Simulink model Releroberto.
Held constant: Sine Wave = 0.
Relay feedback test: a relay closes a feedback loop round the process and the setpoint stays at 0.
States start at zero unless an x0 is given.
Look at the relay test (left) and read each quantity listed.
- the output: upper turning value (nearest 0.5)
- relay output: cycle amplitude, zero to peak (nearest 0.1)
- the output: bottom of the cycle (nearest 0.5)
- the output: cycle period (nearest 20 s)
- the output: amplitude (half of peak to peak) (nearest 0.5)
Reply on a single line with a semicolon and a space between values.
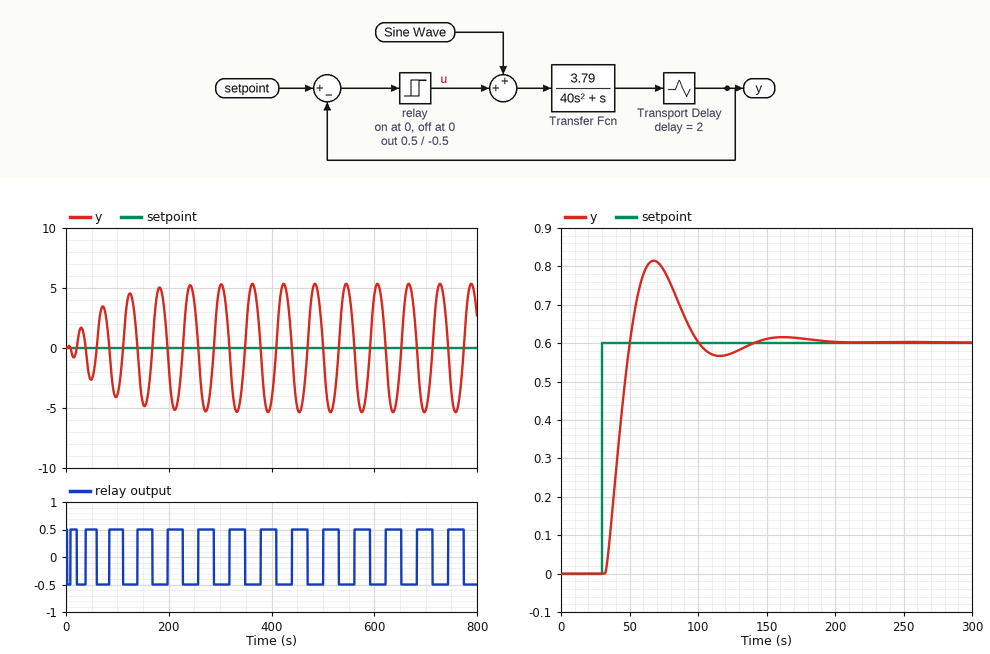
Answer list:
5.5; 0.5; -5.5; 60 s; 5.5
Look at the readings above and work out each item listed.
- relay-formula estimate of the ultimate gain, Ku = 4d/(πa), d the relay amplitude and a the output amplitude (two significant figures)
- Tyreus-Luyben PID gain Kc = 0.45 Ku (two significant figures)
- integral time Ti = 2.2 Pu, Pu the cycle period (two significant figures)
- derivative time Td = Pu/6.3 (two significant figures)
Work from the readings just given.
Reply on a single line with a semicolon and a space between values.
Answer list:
0.12; 0.054; 130 s; 9.5 s
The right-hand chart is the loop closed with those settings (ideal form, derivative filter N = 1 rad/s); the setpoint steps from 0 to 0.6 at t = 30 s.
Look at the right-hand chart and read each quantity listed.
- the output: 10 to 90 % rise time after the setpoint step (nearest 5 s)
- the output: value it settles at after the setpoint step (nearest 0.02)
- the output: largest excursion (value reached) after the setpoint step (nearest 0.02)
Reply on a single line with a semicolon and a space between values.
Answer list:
15 s; 0.60; 0.82
